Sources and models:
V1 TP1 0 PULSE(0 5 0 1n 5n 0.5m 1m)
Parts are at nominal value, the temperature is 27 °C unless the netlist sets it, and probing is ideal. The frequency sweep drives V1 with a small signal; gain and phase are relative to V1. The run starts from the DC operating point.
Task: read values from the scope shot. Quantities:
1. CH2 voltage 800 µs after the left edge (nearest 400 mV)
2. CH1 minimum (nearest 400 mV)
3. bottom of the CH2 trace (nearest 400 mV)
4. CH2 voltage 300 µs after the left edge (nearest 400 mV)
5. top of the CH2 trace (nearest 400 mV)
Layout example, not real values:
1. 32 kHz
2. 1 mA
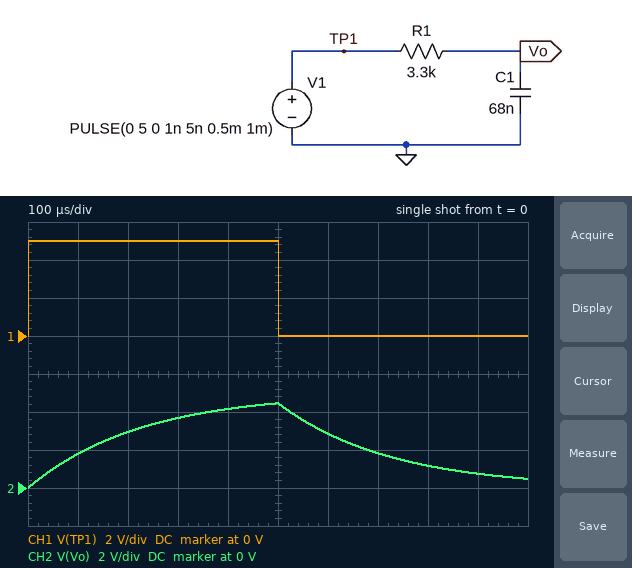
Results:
1. 1.2 V
2. 0 V
3. 0 V
4. 3.6 V
5. 4.4 V
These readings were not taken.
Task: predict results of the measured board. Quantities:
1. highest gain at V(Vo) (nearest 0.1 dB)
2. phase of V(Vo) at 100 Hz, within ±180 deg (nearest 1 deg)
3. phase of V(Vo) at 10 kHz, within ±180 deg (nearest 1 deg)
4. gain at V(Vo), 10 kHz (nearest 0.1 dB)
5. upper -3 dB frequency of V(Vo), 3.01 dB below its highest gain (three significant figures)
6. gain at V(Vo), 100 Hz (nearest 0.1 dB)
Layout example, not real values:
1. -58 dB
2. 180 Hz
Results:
1. 0 dB
2. -8 deg
3. -86 deg
4. -23.0 dB
5. 709 Hz
6. -0.1 dB
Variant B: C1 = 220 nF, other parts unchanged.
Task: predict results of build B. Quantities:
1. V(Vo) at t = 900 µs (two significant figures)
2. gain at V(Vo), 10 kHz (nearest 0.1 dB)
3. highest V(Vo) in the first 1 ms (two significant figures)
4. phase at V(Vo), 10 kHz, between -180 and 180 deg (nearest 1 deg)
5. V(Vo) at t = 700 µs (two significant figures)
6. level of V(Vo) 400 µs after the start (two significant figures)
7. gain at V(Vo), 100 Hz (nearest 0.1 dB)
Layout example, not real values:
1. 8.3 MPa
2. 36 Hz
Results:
1. 1.4 V
2. -33.2 dB
3. 2.5 V
4. -89 deg
5. 1.9 V
6. 2.1 V
7. -0.8 dB
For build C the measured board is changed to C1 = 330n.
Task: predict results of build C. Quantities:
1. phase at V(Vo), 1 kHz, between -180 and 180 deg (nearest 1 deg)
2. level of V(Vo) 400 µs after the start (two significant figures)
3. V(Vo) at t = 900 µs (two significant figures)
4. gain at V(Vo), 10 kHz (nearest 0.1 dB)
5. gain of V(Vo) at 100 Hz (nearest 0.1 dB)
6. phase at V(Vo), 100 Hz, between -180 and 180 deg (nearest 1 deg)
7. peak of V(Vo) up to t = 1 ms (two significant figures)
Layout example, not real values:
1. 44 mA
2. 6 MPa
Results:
1. -82 deg
2. 1.5 V
3. 1.3 V
4. -36.7 dB
5. -1.7 dB
6. -34 deg
7. 1.8 V
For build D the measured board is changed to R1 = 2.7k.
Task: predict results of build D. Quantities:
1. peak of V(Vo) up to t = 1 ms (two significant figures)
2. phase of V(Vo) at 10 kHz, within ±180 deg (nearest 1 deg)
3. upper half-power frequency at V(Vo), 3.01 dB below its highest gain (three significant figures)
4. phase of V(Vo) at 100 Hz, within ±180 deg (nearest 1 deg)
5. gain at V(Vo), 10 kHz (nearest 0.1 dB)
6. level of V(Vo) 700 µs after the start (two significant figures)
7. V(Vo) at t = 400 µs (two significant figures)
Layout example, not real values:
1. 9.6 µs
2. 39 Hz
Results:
1. 4.7 V
2. -85 deg
3. 867 Hz
4. -7 deg
5. -21.3 dB
6. 1.6 V
7. 4.4 V
